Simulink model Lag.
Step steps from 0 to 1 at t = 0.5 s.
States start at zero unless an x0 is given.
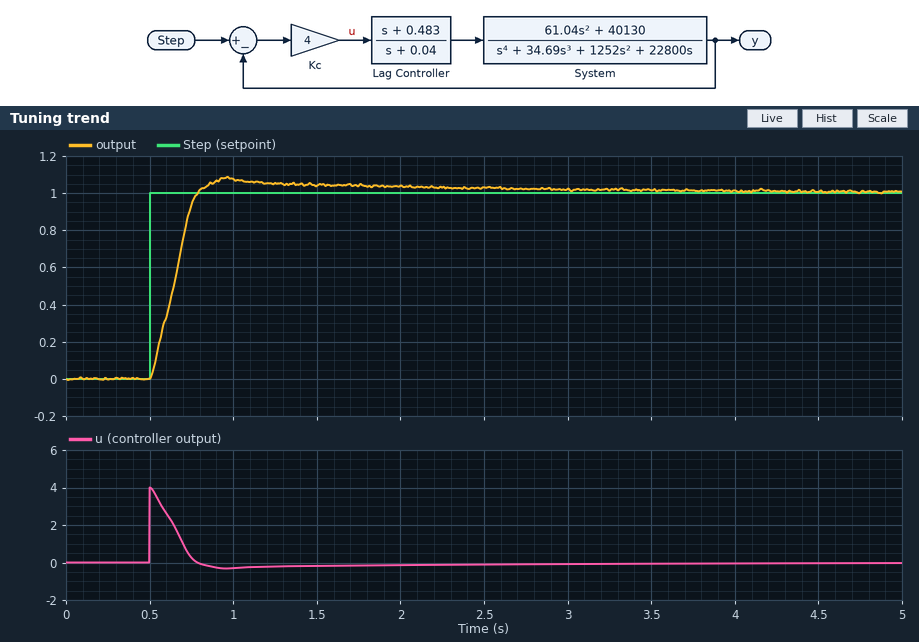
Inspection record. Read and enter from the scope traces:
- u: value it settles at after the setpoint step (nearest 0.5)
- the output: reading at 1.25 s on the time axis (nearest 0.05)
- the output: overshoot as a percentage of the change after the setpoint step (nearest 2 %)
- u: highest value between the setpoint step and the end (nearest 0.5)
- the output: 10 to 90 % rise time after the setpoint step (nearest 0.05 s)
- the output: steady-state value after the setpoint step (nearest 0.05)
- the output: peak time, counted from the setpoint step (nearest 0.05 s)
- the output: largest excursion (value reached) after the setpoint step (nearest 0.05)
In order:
0.0
1.05
8 %
4.0
0.20 s
1.00
0.45 s
1.10
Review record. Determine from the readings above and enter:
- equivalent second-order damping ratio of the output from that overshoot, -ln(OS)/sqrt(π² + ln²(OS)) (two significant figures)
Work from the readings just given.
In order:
0.63
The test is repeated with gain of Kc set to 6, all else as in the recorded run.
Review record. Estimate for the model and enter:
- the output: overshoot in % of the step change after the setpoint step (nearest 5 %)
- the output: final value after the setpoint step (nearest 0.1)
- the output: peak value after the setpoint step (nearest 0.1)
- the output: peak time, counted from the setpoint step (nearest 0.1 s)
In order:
15 %
1.0
1.2
0.3 s
